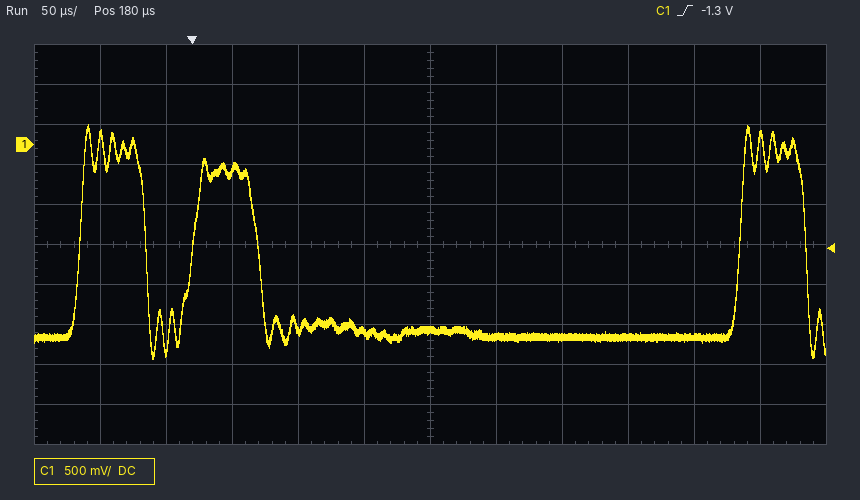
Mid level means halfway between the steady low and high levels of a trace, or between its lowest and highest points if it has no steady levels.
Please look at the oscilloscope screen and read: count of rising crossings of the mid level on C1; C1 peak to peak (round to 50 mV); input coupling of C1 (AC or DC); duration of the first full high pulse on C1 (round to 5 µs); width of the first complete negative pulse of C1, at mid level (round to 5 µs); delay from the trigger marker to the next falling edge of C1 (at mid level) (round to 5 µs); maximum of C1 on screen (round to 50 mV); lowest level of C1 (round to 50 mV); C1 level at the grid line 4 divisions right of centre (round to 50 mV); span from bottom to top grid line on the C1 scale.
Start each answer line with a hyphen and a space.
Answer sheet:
- 3
- 2.95 V
- DC
- 50 µs
- 35 µs
- 50 µs
- 250 mV
- -2.70 V
- -2.40 V
- 5 V
